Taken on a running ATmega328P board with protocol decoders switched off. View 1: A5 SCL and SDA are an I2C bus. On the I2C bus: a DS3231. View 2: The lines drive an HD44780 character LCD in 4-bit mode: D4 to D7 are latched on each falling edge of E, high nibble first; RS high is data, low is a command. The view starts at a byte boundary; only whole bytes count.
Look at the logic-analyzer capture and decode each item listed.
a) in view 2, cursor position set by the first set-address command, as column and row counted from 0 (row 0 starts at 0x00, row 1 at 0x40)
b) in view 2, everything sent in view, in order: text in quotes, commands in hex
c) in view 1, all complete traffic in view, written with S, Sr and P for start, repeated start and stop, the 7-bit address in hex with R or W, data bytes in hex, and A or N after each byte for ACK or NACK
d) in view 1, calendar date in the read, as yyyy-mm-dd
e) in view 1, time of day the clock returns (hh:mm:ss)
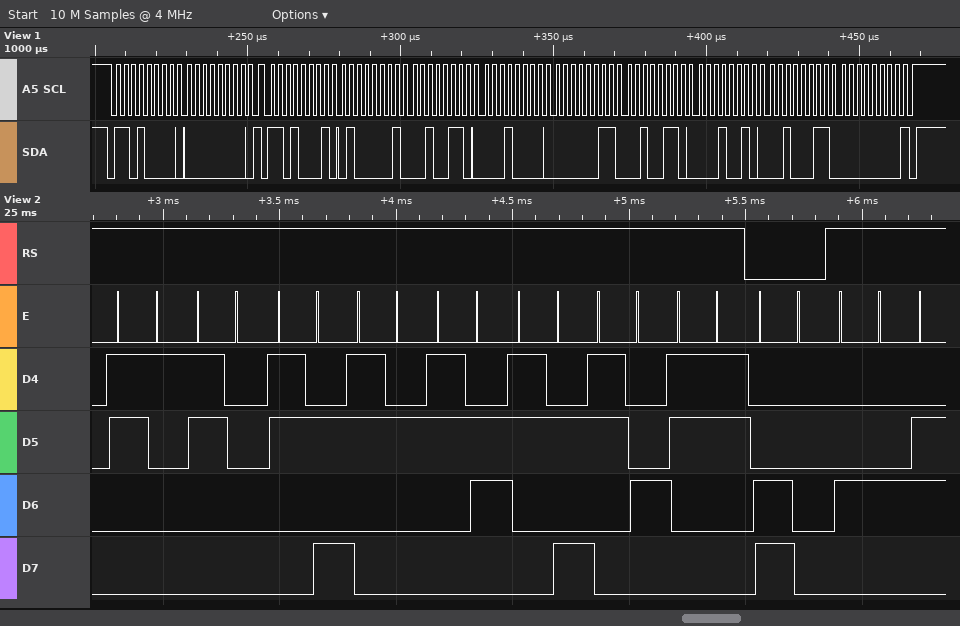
column 0, row 1
"10:26:43" 0xC0 "D"
S 68W A 00 A Sr 68R A 41 A 26 A 10 A 03 A 26 A 12 A 23 A 00 N P
2023-12-26
10:26:41
